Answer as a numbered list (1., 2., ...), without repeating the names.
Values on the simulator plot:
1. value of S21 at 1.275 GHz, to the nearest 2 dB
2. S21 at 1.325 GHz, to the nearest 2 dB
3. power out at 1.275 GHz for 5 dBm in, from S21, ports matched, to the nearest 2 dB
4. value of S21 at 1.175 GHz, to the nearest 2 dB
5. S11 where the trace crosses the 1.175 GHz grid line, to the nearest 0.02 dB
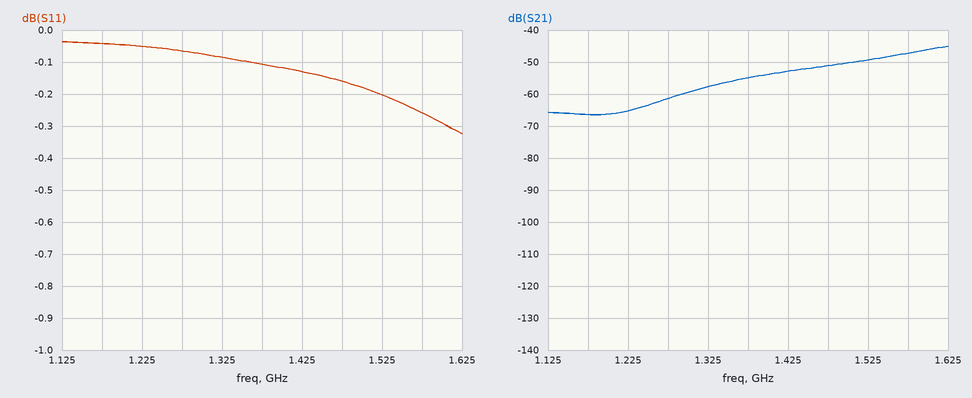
1. -62 dB
2. -58 dB
3. -56 dBm
4. -66 dB
5. -0.04 dB
